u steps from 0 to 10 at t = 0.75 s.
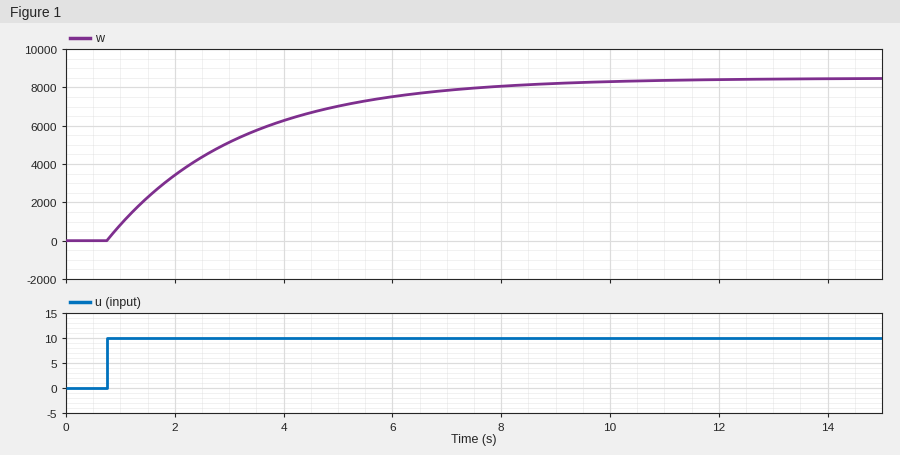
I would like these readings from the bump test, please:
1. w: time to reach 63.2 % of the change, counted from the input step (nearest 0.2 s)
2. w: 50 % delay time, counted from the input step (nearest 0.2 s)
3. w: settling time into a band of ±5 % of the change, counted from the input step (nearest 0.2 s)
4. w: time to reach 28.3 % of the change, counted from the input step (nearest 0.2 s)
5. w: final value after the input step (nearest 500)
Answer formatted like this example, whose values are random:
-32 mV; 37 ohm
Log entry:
2.4 s; 1.6 s; 7.2 s; 0.8 s; 8500
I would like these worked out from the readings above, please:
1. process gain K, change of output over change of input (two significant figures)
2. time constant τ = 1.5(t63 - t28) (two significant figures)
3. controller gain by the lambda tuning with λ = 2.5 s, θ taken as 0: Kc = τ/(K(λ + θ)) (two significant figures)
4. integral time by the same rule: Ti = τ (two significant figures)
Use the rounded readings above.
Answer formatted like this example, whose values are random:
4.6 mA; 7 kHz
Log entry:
850; 2.4 s; 0.0011; 2.4 s
